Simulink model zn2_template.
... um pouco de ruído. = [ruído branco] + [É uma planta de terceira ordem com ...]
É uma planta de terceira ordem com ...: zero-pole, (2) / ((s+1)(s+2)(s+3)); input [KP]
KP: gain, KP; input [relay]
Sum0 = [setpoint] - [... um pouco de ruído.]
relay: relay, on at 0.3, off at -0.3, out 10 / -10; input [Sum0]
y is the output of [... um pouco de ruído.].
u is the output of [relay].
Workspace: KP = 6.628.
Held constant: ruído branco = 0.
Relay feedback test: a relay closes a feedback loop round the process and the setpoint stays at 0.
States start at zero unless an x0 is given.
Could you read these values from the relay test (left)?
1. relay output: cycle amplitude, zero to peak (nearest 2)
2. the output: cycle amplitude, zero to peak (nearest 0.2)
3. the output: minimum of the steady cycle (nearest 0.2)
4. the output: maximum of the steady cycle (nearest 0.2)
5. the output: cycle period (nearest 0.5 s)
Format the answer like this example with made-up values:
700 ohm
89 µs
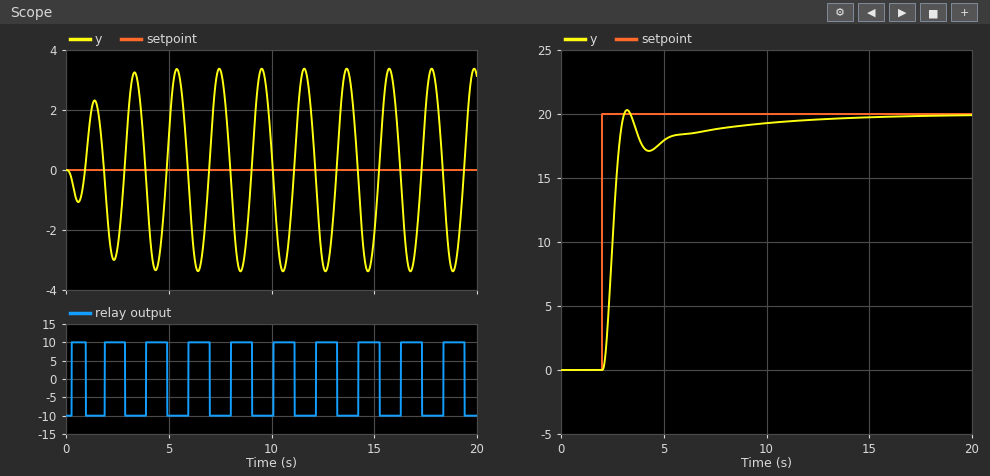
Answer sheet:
10
3.4
-3.4
3.4
2.0 s
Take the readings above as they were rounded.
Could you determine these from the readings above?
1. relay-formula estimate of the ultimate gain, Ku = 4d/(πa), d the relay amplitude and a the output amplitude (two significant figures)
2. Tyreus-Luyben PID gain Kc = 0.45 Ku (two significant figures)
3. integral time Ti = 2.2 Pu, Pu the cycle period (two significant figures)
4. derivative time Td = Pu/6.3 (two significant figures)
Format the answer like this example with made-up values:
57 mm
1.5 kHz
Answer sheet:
3.7
1.7
4.4 s
0.32 s
